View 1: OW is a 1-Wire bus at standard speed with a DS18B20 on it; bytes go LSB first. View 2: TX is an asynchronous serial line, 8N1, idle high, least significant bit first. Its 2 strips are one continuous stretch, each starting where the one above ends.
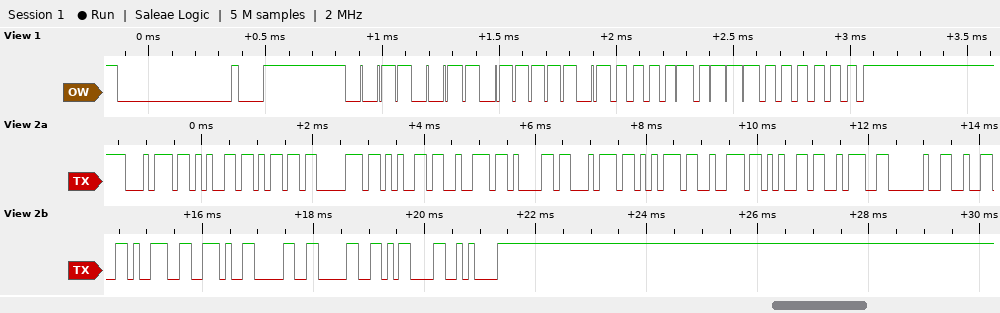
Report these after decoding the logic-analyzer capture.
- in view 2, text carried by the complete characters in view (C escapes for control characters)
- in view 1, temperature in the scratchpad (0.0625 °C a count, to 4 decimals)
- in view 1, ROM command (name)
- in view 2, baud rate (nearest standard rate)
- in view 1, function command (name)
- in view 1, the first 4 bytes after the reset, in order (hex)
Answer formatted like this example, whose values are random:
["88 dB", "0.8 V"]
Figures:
["\"temperature: 29.00\\r\\n\"", "29.0000 °C", "Skip ROM", "9600 baud", "Read Scratchpad", "CC BE D0 01"]
